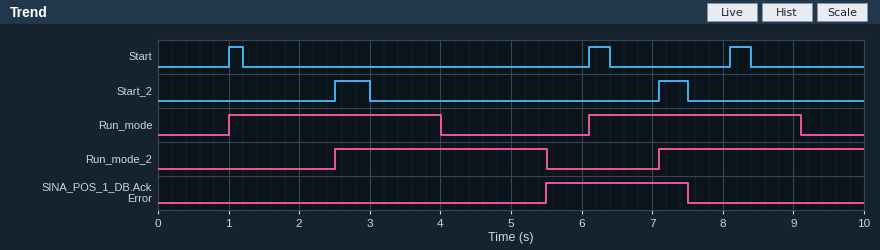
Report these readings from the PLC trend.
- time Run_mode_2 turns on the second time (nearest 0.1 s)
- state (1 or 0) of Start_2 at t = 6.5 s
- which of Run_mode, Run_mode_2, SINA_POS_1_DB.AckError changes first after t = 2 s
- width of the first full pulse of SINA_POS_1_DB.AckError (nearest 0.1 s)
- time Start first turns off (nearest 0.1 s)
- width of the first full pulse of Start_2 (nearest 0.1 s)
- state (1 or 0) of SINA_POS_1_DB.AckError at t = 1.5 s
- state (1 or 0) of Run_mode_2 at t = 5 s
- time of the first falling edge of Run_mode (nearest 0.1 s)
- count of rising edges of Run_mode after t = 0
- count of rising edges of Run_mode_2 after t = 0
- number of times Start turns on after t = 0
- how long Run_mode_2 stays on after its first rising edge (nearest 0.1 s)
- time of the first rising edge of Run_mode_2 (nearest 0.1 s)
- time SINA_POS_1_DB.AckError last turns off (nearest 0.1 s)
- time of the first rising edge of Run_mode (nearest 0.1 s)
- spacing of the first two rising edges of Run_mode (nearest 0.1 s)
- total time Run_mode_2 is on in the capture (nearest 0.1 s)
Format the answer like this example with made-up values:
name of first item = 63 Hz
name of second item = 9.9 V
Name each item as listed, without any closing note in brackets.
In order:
time Run_mode_2 turns on the second time = 7.1 s
state (1 or 0) of Start_2 at t = 6.5 s = 0
which of Run_mode, Run_mode_2, SINA_POS_1_DB.AckError changes first after t = 2 s = Run_mode_2
width of the first full pulse of SINA_POS_1_DB.AckError = 2.0 s
time Start first turns off = 1.2 s
width of the first full pulse of Start_2 = 0.5 s
state (1 or 0) of SINA_POS_1_DB.AckError at t = 1.5 s = 0
state (1 or 0) of Run_mode_2 at t = 5 s = 1
time of the first falling edge of Run_mode = 4.0 s
count of rising edges of Run_mode after t = 0 = 2
count of rising edges of Run_mode_2 after t = 0 = 2
number of times Start turns on after t = 0 = 3
how long Run_mode_2 stays on after its first rising edge = 3.0 s
time of the first rising edge of Run_mode_2 = 2.5 s
time SINA_POS_1_DB.AckError last turns off = 7.5 s
time of the first rising edge of Run_mode = 1.0 s
spacing of the first two rising edges of Run_mode = 5.1 s
total time Run_mode_2 is on in the capture = 5.9 s
